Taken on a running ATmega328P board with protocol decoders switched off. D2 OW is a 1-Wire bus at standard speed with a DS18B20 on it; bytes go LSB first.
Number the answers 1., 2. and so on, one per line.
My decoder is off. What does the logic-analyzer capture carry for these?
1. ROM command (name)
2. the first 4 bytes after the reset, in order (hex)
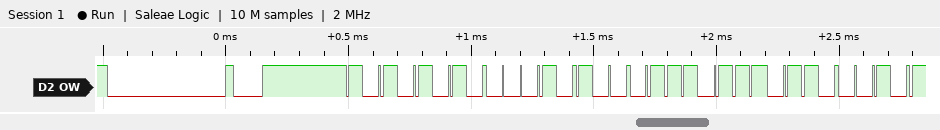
1. Match ROM
2. 55 28 EE 46
